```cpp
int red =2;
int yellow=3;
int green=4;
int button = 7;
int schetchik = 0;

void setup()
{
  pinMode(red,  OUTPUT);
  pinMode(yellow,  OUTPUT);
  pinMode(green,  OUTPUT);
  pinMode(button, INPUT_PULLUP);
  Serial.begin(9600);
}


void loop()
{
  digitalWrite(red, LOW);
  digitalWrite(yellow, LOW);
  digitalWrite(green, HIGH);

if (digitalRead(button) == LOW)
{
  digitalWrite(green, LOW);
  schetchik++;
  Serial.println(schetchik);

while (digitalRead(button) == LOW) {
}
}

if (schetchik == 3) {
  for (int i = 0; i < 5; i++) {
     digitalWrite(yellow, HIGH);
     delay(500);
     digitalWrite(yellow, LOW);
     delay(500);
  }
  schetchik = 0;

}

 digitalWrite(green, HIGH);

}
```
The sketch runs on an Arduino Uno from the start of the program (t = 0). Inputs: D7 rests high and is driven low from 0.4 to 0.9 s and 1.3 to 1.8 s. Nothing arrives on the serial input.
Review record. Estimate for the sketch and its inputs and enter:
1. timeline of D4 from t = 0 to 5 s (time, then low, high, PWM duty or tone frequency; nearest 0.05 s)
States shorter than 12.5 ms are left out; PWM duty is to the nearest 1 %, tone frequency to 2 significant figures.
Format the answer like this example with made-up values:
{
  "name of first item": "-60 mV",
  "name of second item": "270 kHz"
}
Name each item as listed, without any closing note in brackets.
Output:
{
  "timeline of D4 from t = 0 to 5 s": "0 s high; 0.4 s low; 0.9 s high; 1.3 s low; 1.8 s high"
}
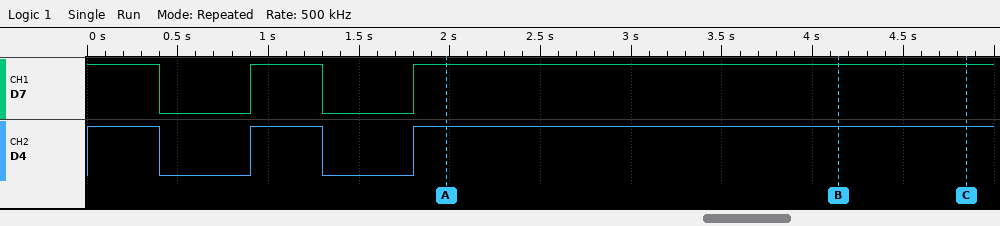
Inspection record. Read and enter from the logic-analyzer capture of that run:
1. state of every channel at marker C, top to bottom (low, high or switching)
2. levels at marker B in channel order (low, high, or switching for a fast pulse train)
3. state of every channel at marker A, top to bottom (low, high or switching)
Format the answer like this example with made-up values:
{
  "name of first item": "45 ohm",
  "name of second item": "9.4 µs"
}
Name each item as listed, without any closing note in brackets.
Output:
{
  "state of every channel at marker C, top to bottom": "D7 high, D4 high",
  "levels at marker B in channel order": "D7 high, D4 high",
  "state of every channel at marker A, top to bottom": "D7 high, D4 high"
}
